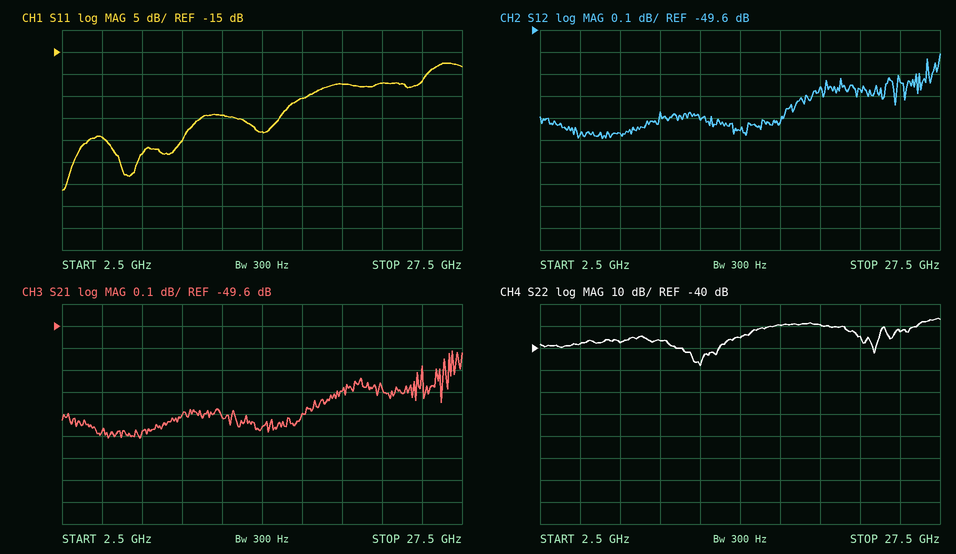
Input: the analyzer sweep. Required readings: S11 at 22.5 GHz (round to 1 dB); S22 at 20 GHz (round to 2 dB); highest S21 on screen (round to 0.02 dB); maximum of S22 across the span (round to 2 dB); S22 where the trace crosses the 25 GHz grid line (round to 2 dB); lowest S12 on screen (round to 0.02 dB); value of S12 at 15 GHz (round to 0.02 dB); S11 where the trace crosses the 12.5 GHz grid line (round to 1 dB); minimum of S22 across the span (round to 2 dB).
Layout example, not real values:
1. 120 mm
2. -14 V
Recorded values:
1. -22 dB
2. -30 dB
3. -49.72 dB
4. -26 dB
5. -32 dB
6. -50.10 dB
7. -50.06 dB
8. -29 dB
9. -48 dB
